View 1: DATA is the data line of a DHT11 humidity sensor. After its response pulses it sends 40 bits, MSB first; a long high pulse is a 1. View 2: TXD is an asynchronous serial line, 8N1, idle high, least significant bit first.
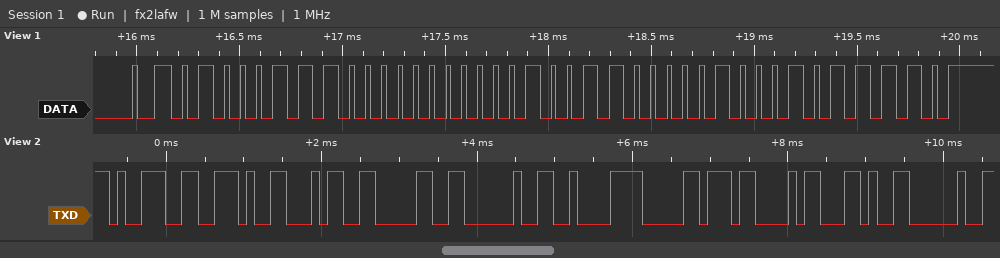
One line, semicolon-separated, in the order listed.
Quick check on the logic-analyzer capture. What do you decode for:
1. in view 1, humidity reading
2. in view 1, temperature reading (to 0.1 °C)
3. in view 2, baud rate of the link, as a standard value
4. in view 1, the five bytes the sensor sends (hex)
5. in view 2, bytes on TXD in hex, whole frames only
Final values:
71 %; 19.4 °C; 9600 baud; 47 00 13 04 5E; 39 2E 34 30 20 C2 B0 43 2C 20
